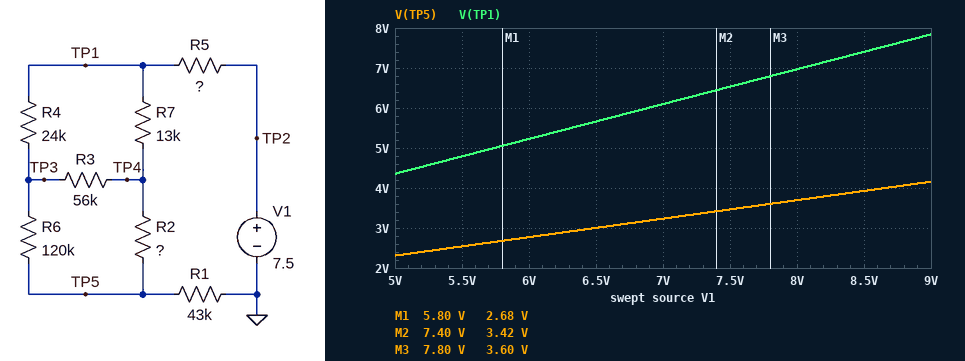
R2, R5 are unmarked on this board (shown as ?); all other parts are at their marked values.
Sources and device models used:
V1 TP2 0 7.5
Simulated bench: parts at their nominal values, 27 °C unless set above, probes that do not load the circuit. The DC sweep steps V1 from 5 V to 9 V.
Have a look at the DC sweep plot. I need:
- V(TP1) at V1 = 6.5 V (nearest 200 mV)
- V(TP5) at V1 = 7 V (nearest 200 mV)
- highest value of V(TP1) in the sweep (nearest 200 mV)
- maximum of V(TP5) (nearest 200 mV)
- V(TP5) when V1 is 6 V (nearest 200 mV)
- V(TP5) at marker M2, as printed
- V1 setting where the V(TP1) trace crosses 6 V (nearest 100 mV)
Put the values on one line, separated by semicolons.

5.6 V; 3.2 V; 7.8 V; 4.2 V; 2.8 V; 3.42 V; 6.9 V
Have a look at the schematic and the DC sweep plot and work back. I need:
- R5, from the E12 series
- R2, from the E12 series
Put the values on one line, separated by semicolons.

12 kΩ; 39 kΩ
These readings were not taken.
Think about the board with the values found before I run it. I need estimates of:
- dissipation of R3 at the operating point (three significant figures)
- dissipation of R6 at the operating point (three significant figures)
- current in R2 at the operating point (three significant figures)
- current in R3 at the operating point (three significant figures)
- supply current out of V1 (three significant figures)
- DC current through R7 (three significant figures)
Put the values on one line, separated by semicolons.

498 nW; 52.0 µW; 59.8 µA; 2.98 µA; 80.6 µA; 56.8 µA
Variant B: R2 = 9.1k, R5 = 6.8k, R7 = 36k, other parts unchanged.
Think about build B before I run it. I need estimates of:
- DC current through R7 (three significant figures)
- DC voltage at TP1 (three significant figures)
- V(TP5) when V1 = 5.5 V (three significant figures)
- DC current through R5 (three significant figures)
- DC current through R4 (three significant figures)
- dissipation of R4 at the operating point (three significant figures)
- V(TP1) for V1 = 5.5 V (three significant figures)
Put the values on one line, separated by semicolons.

57.6 µA; 6.86 V; 2.98 V; 94.6 µA; 37.0 µA; 32.9 µW; 5.03 V
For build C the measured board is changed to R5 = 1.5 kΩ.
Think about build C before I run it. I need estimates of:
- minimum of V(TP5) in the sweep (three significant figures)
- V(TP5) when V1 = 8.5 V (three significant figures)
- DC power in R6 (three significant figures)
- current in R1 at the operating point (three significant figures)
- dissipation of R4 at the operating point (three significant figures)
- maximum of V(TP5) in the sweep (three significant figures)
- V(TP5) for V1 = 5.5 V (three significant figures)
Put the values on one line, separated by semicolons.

2.60 V; 4.43 V; 66.0 µW; 90.8 µA; 17.3 µW; 4.69 V; 2.86 V
